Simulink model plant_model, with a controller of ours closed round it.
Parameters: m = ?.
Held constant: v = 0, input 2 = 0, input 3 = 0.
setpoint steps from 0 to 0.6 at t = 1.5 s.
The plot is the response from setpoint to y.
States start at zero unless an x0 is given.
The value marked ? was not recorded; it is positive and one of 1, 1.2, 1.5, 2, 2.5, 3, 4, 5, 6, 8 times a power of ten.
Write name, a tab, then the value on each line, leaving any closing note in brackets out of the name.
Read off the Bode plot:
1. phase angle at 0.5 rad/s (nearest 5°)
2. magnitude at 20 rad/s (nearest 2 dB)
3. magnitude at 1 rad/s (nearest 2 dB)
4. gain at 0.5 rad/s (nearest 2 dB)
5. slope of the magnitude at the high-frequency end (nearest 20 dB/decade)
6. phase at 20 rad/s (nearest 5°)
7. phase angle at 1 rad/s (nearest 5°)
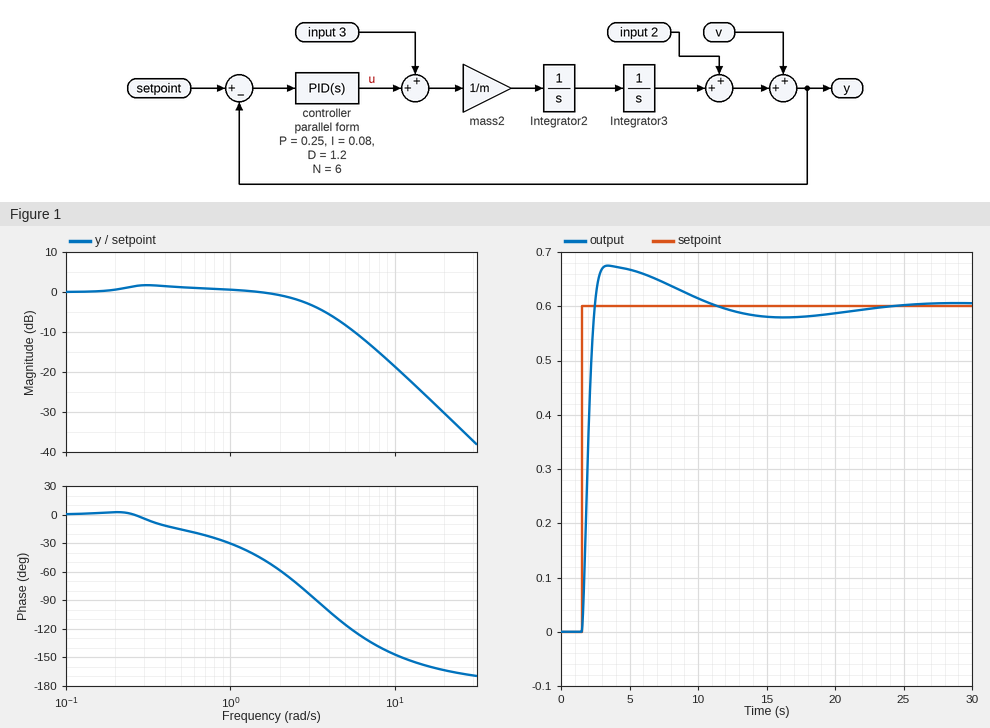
phase angle at 0.5 rad/s	-15°
magnitude at 20 rad/s	-30 dB
magnitude at 1 rad/s	0 dB
gain at 0.5 rad/s	2 dB
slope of the magnitude at the high-frequency end	-40 dB/decade
phase at 20 rad/s	-165°
phase angle at 1 rad/s	-30°
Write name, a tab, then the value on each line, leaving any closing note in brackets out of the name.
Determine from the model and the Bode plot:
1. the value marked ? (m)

the value marked ?	0.6
